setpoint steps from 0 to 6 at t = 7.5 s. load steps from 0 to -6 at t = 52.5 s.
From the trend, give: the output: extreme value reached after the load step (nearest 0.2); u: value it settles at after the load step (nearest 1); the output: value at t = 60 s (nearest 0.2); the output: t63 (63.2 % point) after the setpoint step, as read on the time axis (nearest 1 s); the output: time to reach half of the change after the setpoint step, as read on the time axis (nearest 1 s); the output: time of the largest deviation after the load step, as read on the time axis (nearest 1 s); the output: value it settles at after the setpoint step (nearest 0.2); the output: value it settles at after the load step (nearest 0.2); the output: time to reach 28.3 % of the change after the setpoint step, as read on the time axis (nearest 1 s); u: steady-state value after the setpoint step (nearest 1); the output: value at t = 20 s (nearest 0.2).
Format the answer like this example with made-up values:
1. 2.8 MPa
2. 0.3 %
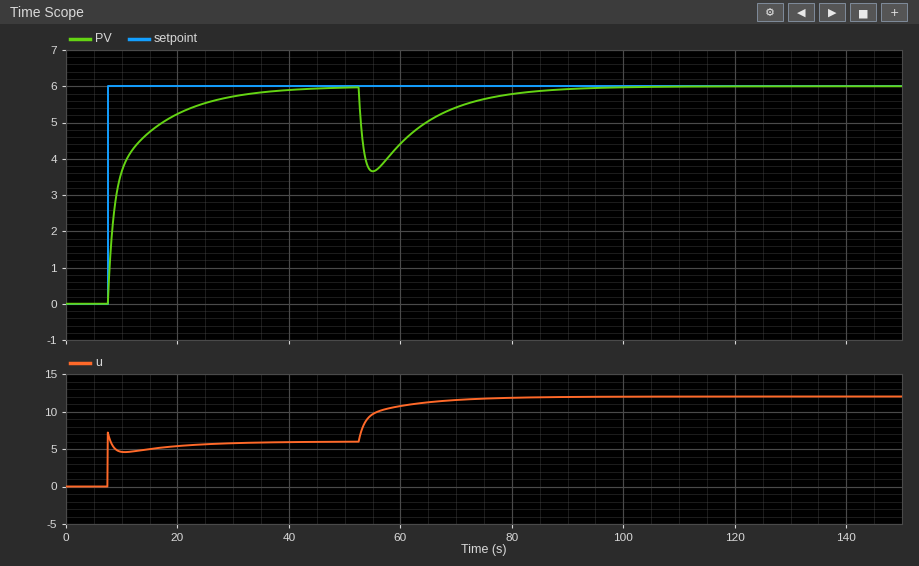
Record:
1. 3.6
2. 12
3. 4.4
4. 10 s
5. 9 s
6. 55 s
7. 6.0
8. 6.0
9. 8 s
10. 6
11. 5.2
